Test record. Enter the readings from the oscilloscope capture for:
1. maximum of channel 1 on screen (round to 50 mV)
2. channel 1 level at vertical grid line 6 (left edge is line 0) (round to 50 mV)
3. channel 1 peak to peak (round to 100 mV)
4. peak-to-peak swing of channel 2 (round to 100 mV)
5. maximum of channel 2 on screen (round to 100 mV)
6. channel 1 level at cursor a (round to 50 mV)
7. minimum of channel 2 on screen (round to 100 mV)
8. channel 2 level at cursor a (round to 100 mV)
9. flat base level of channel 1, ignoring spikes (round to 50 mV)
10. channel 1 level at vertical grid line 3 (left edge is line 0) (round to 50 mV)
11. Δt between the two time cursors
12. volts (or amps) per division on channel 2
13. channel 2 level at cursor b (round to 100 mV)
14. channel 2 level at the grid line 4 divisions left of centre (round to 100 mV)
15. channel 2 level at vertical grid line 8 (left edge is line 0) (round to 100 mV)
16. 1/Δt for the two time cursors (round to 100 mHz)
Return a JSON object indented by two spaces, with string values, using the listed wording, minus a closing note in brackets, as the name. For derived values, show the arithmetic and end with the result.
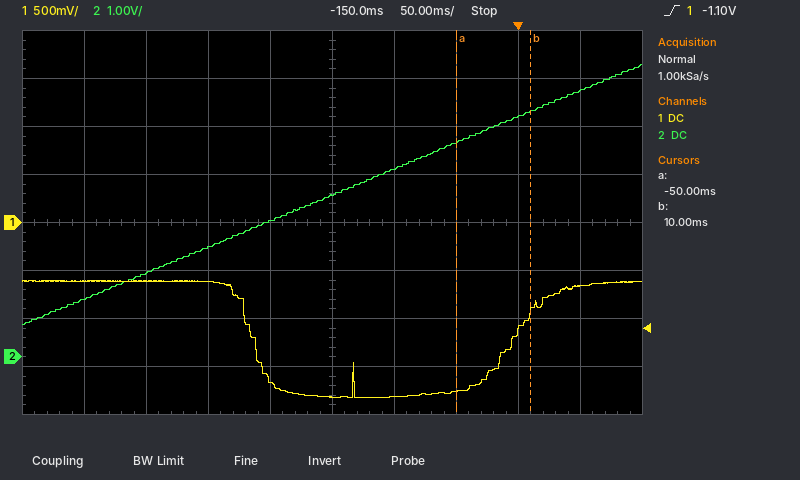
{
  "maximum of channel 1 on screen": "-600 mV",
  "channel 1 level at vertical grid line 6 (left edge is line 0)": "-1.80 V",
  "channel 1 peak to peak": "1.20 V",
  "peak-to-peak swing of channel 2": "6.1 V − (700 mV) = 5.4 V",
  "maximum of channel 2 on screen": "6.1 V",
  "channel 1 level at cursor a": "-1.75 V",
  "minimum of channel 2 on screen": "700 mV",
  "channel 2 level at cursor a": "4.5 V",
  "flat base level of channel 1, ignoring spikes": "-1.80 V",
  "channel 1 level at vertical grid line 3 (left edge is line 0)": "-600 mV",
  "Δt between the two time cursors": "10 ms − (-50 ms) = 60 ms",
  "volts (or amps) per division on channel 2": "1 V",
  "channel 2 level at cursor b": "5.1 V",
  "channel 2 level at the grid line 4 divisions left of centre": "1.2 V",
  "channel 2 level at vertical grid line 8 (left edge is line 0)": "5.0 V",
  "1/Δt for the two time cursors": "1 / 60 ms ≈ 16.7 Hz"
}
